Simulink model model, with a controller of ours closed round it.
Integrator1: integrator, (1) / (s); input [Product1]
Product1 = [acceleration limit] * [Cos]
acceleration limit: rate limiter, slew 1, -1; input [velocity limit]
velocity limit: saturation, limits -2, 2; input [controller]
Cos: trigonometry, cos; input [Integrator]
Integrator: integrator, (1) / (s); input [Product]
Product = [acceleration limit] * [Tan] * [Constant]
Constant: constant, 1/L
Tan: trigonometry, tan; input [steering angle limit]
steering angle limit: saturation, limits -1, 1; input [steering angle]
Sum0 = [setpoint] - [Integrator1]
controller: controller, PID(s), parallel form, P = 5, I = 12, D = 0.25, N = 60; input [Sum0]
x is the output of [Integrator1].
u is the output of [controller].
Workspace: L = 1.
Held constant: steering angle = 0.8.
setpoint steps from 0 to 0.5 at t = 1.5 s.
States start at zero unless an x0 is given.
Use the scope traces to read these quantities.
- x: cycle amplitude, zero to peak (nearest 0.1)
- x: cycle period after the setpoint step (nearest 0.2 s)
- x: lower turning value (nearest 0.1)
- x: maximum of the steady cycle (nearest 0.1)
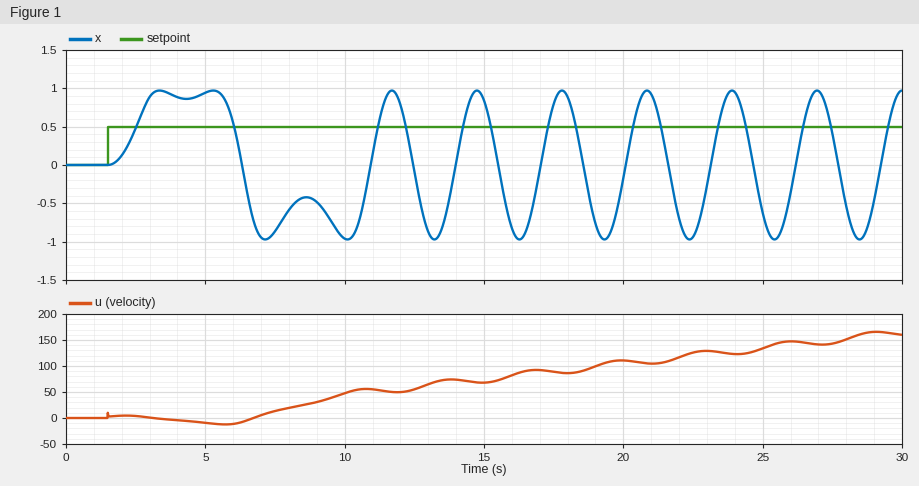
1.0
3.0 s
-1.0
1.0
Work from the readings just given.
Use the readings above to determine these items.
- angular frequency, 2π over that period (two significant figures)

2.1 rad/s
